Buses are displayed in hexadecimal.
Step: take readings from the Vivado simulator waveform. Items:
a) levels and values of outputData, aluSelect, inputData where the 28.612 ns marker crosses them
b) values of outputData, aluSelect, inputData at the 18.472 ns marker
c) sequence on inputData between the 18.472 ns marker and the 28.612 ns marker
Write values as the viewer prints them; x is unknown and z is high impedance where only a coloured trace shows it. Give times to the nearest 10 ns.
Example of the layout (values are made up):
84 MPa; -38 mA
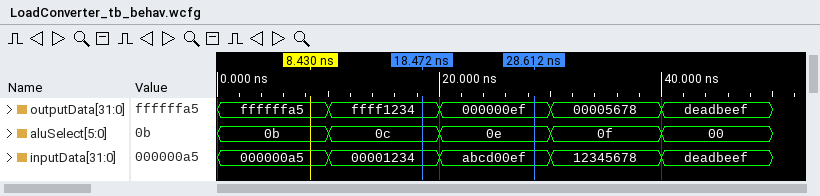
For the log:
outputData=000000ef, aluSelect=0e, inputData=abcd00ef; outputData=ffff1234, aluSelect=0c, inputData=00001234; 00001234, abcd00ef
